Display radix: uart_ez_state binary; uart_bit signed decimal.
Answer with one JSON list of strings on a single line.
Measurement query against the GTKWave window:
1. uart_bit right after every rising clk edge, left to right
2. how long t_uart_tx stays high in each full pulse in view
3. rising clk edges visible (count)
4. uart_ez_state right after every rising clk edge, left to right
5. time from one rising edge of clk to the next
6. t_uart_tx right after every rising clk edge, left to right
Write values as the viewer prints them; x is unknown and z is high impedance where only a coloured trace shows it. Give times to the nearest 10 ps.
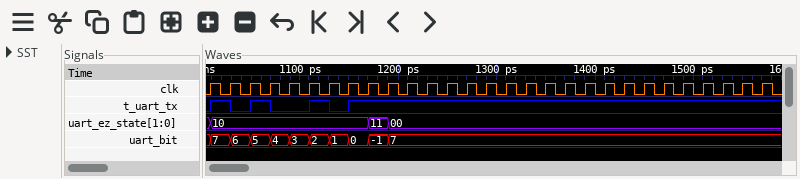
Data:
["7, 6, 5, 4, 3, 2, 1, 0, -1, 7, 7, 7, 7, 7, 7, 7, 7, 7, 7, 7, 7, 7, 7, 7, 7, 7, 7, 7, 7", "20 ps, 20 ps, 20 ps", "29", "10, 10, 10, 10, 10, 10, 10, 10, 11, 00, 00, 00, 00, 00, 00, 00, 00, 00, 00, 00, 00, 00, 00, 00, 00, 00, 00, 00, 00", "20 ps", "1 0 1 0 0 1 0 1 1 1 1 1 1 1 1 1 1 1 1 1 1 1 1 1 1 1 1 1 1"]
